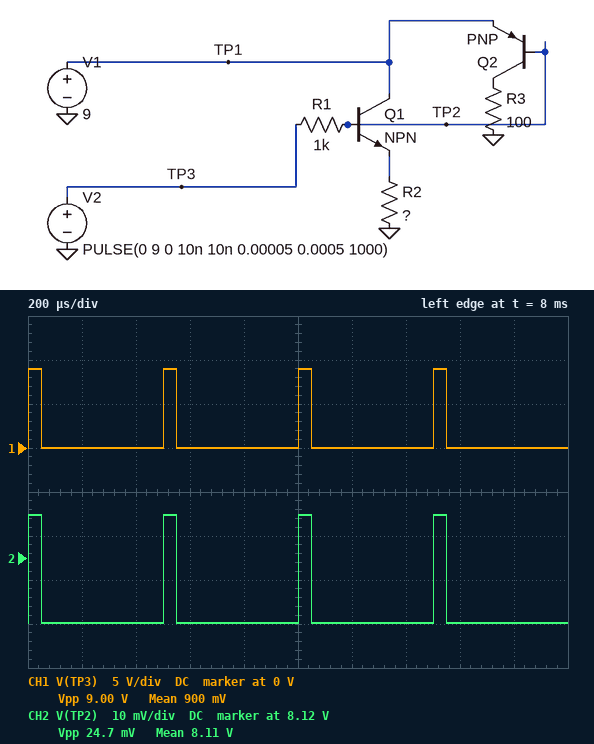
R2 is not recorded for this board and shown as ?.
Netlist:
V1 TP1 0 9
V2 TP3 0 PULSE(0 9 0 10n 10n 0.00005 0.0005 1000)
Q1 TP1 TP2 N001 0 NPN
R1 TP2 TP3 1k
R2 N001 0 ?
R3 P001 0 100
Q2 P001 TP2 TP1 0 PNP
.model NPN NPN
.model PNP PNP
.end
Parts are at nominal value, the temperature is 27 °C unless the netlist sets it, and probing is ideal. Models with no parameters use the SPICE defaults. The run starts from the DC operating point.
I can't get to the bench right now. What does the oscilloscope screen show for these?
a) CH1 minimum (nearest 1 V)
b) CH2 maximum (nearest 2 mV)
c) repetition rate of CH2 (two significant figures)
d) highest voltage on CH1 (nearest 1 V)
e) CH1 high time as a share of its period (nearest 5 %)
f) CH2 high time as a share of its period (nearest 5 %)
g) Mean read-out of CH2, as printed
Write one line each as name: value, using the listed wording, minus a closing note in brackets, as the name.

CH1 minimum: 0 V
CH2 maximum: 8.130 V
repetition rate of CH2: 2.0 kHz
highest voltage on CH1: 9 V
CH1 high time as a share of its period: 10 %
CH2 high time as a share of its period: 10 %
Mean read-out of CH2, as printed: 8.11 V
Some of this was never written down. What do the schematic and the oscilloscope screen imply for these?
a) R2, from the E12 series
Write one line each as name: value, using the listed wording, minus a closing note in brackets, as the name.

R2, from the E12 series: 56 Ω
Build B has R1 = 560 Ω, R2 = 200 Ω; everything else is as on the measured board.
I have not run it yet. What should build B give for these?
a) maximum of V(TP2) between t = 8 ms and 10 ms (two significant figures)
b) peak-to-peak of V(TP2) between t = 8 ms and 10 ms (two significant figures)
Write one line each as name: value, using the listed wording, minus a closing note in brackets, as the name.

maximum of V(TP2) between t = 8 ms and 10 ms: 8.8 V
peak-to-peak of V(TP2) between t = 8 ms and 10 ms: 680 mV
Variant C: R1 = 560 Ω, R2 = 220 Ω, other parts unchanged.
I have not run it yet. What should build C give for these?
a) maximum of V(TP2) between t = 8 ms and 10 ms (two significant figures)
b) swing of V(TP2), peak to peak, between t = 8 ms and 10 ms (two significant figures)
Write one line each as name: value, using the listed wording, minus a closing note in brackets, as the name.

maximum of V(TP2) between t = 8 ms and 10 ms: 8.8 V
swing of V(TP2), peak to peak, between t = 8 ms and 10 ms: 700 mV
